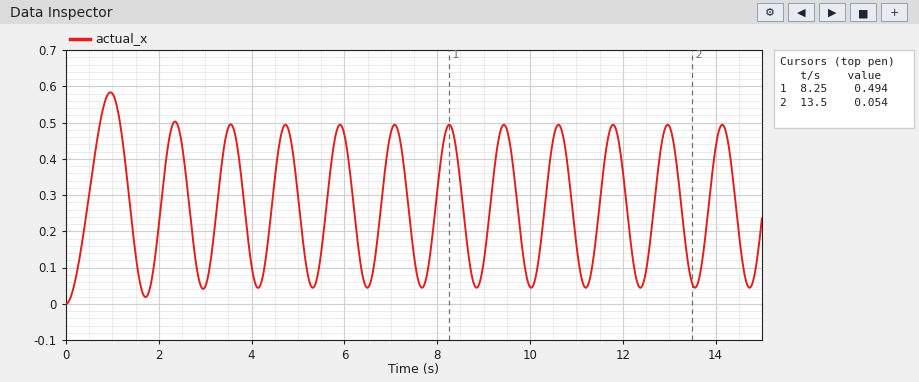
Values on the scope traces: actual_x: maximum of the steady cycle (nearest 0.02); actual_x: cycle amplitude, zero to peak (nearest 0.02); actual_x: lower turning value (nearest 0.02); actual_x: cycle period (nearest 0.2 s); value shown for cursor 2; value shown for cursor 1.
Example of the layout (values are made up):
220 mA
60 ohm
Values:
0.50
0.22
0.04
1.2 s
0.054
0.494
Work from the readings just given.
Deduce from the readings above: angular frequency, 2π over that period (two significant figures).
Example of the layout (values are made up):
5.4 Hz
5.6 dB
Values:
5.2 rad/s
